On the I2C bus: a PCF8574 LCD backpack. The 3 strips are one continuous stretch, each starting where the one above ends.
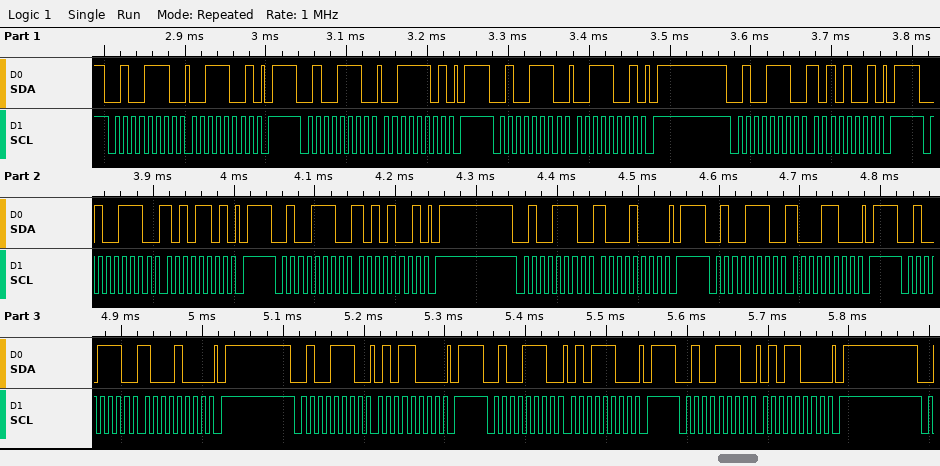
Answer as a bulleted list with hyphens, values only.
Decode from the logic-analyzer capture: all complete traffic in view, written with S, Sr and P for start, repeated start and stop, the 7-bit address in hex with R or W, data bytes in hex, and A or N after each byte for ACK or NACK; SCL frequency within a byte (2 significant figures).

- S 27W A 39 A P S 27W A 3D A P S 27W A 39 A P S 27W A A9 A P S 27W A AD A P S 27W A A9 A P S 27W A 88 A P S 27W A 8C A P S 27W A 88 A P S 27W A 58 A P S 27W A 5C A P S 27W A 58 A P
- 100 kHz
